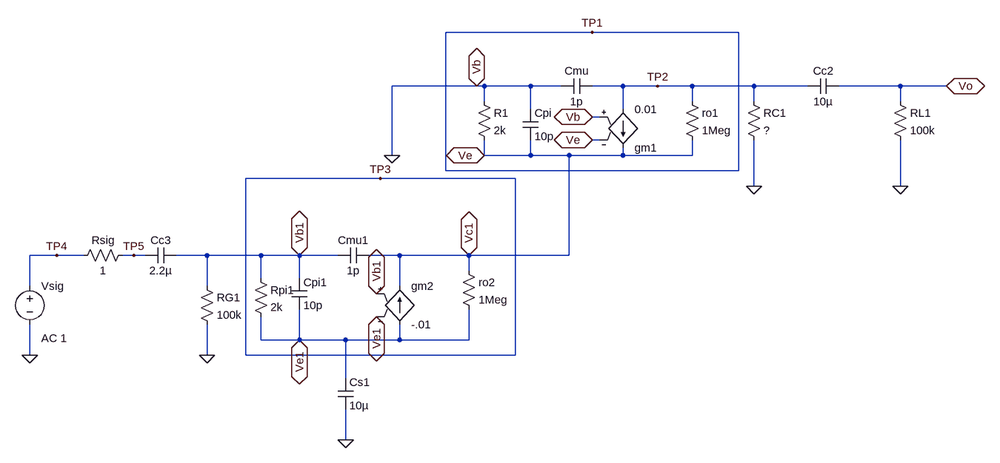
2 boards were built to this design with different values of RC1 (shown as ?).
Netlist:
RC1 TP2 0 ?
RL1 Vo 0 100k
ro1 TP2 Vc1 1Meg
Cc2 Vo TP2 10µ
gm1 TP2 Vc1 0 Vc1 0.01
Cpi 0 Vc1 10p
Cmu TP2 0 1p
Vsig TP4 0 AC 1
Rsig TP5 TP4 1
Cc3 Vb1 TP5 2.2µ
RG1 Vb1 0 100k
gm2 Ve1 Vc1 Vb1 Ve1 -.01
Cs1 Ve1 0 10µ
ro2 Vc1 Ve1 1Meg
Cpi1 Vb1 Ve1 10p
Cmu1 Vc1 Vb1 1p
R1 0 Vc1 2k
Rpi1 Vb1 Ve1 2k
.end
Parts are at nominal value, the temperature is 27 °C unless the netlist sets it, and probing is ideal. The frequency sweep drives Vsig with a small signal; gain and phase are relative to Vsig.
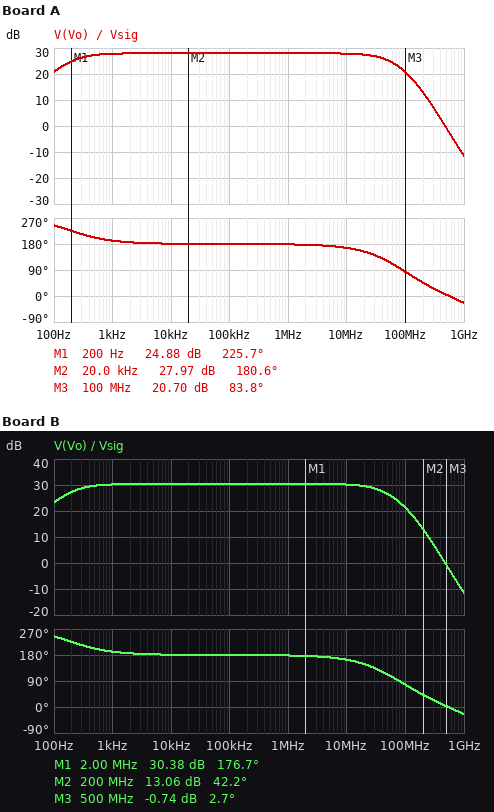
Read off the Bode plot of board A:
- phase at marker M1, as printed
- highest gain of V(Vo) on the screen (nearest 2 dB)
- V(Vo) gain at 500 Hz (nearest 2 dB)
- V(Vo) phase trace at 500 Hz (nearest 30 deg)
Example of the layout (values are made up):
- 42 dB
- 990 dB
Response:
- 225.7 deg
- 28 dB
- 28 dB
- 210 deg
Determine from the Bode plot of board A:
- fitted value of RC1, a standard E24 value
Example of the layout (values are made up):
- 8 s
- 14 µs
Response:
- 2.7 kΩ
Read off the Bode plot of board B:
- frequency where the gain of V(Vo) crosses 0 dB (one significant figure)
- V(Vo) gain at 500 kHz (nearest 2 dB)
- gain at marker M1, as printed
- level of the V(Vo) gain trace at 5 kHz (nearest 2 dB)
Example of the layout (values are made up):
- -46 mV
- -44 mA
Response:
- 500 MHz
- 30 dB
- 30.38 dB
- 30 dB
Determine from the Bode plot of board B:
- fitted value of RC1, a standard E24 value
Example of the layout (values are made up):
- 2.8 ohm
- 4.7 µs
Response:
- 3.6 kΩ
